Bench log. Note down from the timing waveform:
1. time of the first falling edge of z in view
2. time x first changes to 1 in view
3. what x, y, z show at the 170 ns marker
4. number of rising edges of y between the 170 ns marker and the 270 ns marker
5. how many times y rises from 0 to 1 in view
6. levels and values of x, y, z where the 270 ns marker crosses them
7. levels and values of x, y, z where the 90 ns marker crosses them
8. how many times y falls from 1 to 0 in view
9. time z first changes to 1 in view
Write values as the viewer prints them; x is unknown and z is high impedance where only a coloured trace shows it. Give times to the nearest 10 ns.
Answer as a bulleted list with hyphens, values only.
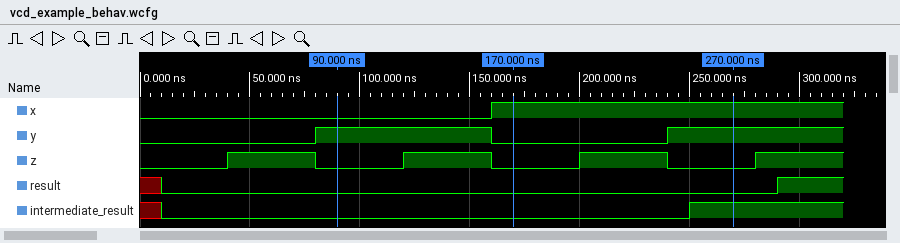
- 80 ns
- 160 ns
- x=1, y=0, z=0
- 1
- 2
- x=1, y=1, z=0
- x=0, y=1, z=0
- 1
- 40 ns
